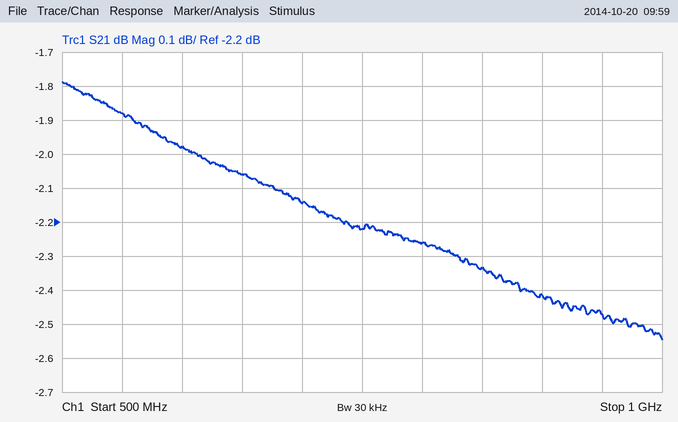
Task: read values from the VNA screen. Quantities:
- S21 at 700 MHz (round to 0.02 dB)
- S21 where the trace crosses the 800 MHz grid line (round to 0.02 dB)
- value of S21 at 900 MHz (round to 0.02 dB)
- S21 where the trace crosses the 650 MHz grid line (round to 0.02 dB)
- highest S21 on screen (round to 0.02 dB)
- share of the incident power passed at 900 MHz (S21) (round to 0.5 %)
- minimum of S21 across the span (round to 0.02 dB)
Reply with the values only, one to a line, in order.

-2.14 dB
-2.26 dB
-2.42 dB
-2.06 dB
-1.78 dB
57.5 %
-2.54 dB
